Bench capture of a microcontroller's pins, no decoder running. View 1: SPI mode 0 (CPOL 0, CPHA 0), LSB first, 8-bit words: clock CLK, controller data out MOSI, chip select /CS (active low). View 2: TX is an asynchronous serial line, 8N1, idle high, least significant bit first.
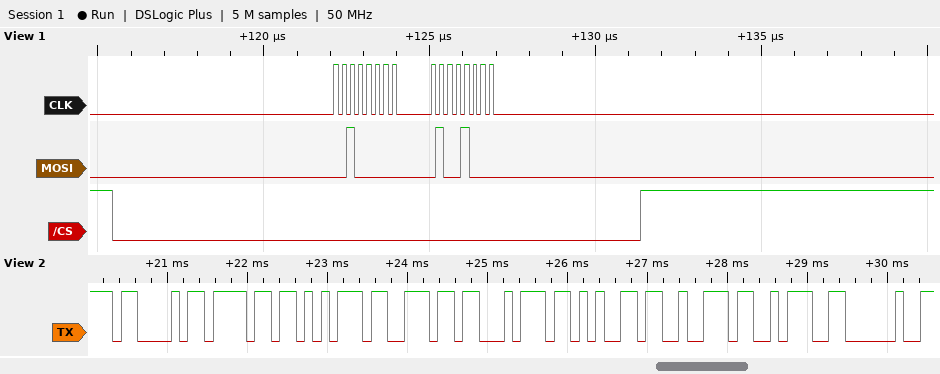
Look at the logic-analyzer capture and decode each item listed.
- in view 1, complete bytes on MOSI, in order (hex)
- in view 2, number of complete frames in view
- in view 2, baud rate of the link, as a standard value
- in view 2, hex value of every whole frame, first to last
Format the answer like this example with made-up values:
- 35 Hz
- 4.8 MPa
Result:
- 04 12
- 9
- 9600 baud
- 43 6F 75 6E 74 65 72 3A 20
